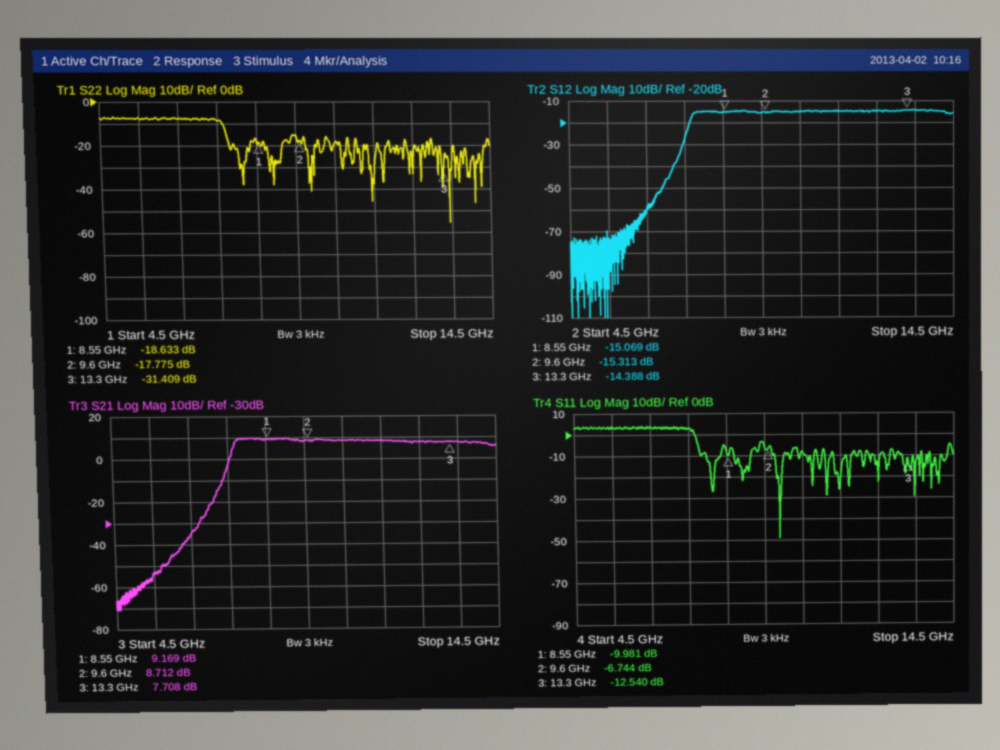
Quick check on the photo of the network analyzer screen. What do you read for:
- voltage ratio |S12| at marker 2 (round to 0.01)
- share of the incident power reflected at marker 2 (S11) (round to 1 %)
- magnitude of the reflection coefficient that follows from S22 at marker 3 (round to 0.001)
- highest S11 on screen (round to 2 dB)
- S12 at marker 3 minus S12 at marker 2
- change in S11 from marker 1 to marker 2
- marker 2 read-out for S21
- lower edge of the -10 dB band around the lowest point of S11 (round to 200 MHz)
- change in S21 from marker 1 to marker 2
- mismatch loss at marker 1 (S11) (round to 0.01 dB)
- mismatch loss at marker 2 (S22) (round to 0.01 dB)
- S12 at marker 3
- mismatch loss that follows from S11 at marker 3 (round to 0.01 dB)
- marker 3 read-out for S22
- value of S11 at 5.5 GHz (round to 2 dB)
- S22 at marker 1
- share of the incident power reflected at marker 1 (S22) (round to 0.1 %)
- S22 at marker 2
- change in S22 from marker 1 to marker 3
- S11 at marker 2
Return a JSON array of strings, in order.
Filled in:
["0.17", "21 %", "0.027", "4 dB", "0.925 dB", "3.237 dB", "8.712 dB", "9.8 GHz", "-0.457 dB", "0.46 dB", "0.07 dB", "-14.388 dB", "0.25 dB", "-31.409 dB", "4 dB", "-18.633 dB", "1.4 %", "-17.775 dB", "-12.776 dB", "-6.744 dB"]
